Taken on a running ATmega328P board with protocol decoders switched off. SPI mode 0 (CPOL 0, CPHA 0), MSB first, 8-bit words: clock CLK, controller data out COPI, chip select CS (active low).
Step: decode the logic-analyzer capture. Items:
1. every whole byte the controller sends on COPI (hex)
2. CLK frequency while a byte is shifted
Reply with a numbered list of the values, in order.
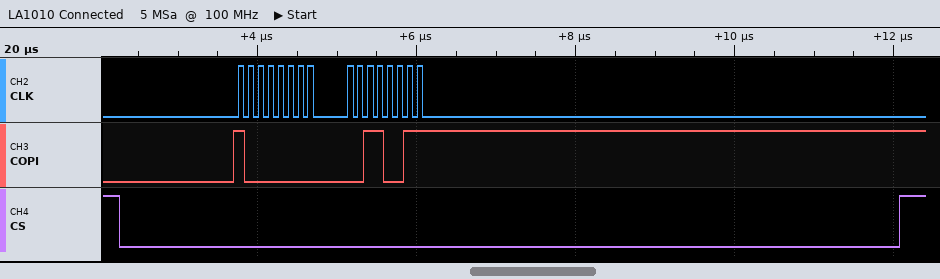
1. 80 33
2. 8 MHz
